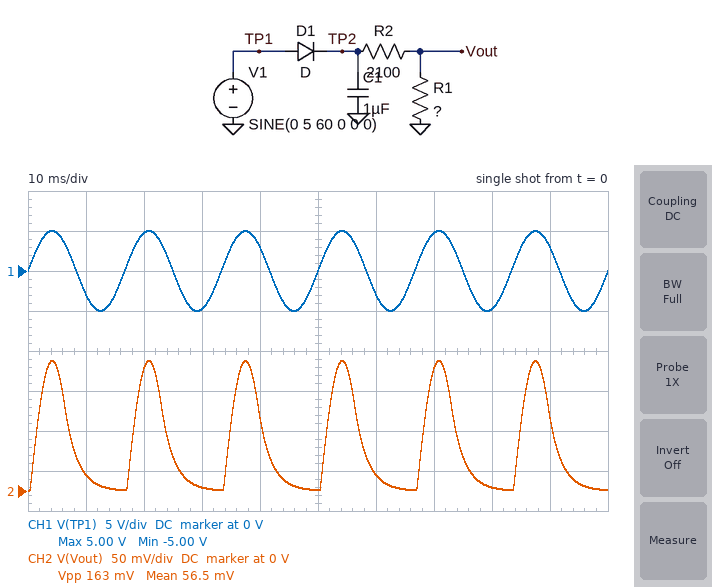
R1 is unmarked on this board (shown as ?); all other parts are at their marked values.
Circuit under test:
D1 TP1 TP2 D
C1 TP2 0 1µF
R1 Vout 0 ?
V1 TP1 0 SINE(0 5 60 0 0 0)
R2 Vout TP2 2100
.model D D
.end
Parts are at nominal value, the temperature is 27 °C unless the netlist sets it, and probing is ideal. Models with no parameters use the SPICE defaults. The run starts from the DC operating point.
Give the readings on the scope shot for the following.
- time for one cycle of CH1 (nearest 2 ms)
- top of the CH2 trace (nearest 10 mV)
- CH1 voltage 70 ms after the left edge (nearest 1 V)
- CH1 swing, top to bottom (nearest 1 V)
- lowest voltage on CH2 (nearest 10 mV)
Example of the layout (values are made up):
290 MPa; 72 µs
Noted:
16 ms; 160 mV; 5 V; 10 V; 0 V
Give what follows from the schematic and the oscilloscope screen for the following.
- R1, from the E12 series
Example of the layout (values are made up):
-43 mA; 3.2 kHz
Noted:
82 Ω
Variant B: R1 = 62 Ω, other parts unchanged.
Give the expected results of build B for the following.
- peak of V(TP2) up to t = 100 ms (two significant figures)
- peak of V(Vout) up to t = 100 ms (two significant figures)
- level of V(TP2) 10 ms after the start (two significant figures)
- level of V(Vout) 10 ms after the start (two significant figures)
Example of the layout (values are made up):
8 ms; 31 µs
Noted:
4.3 V; 120 mV; 520 mV; 15 mV
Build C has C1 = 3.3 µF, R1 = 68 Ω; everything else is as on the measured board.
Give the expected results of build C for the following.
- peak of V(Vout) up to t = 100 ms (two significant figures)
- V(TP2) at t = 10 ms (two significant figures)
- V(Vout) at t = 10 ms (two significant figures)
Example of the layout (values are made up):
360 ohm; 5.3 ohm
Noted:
140 mV; 2.1 V; 65 mV
